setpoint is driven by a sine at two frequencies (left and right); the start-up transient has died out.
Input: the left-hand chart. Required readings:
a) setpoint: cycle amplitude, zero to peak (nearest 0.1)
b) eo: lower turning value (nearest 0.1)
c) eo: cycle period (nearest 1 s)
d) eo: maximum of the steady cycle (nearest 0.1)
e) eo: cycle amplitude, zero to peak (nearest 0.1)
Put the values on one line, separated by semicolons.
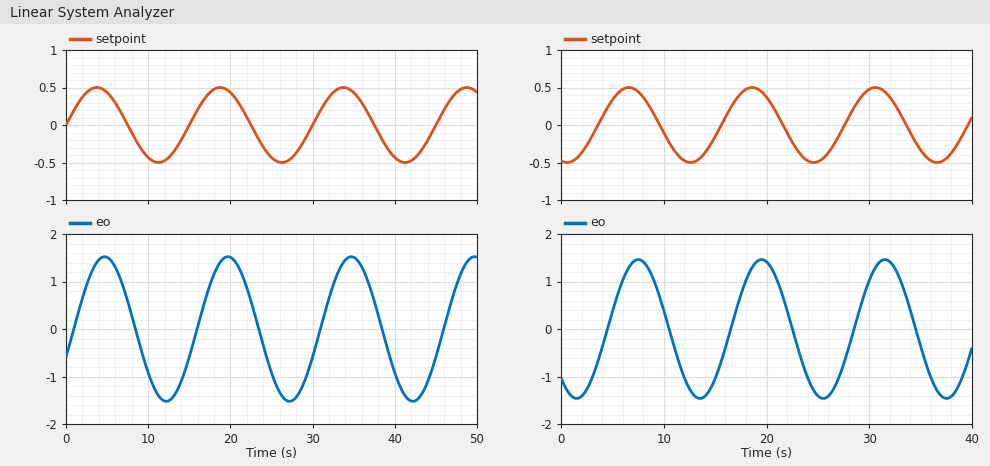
0.5; -1.5; 15 s; 1.5; 1.5
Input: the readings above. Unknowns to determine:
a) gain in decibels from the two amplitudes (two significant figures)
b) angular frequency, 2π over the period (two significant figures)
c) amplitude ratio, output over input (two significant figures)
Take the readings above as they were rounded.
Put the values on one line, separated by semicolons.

9.5 dB; 0.42 rad/s; 3.0
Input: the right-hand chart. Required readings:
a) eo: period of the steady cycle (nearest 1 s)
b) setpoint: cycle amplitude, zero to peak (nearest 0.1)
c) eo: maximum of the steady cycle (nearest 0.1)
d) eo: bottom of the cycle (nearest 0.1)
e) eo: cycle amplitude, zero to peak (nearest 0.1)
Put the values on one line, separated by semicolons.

12 s; 0.5; 1.5; -1.5; 1.5
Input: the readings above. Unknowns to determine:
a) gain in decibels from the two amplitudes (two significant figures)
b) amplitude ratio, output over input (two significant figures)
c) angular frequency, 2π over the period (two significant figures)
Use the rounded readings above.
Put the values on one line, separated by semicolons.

9.5 dB; 3.0; 0.52 rad/s
